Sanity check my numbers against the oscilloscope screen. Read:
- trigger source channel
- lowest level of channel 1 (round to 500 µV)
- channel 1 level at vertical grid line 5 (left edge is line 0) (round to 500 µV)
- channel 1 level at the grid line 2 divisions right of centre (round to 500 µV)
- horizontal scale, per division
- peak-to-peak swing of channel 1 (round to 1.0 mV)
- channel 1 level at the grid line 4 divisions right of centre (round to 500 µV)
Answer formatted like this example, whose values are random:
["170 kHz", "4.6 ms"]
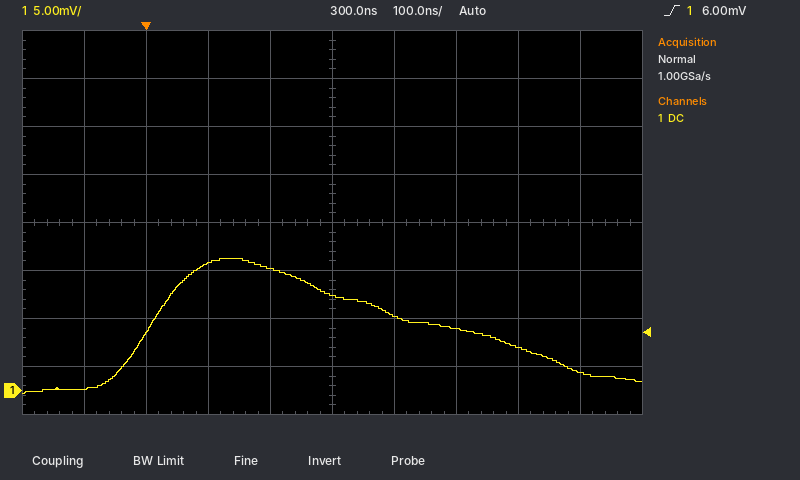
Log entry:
["channel 1", "-500 µV", "10.0 mV", "6.5 mV", "100 ns", "14.0 mV", "2.0 mV"]
